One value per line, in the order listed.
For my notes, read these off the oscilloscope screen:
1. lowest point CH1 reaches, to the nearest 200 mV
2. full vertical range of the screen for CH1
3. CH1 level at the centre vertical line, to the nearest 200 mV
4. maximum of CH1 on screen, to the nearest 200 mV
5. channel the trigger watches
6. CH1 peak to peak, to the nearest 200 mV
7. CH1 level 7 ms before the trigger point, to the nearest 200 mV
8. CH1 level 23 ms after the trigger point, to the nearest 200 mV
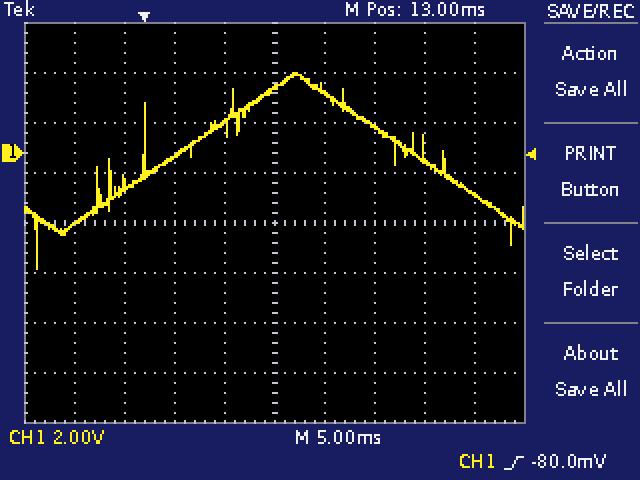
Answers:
-4.6 V
16 V
2.6 V
3.2 V
CH1
7.8 V
-2.8 V
1.0 V
